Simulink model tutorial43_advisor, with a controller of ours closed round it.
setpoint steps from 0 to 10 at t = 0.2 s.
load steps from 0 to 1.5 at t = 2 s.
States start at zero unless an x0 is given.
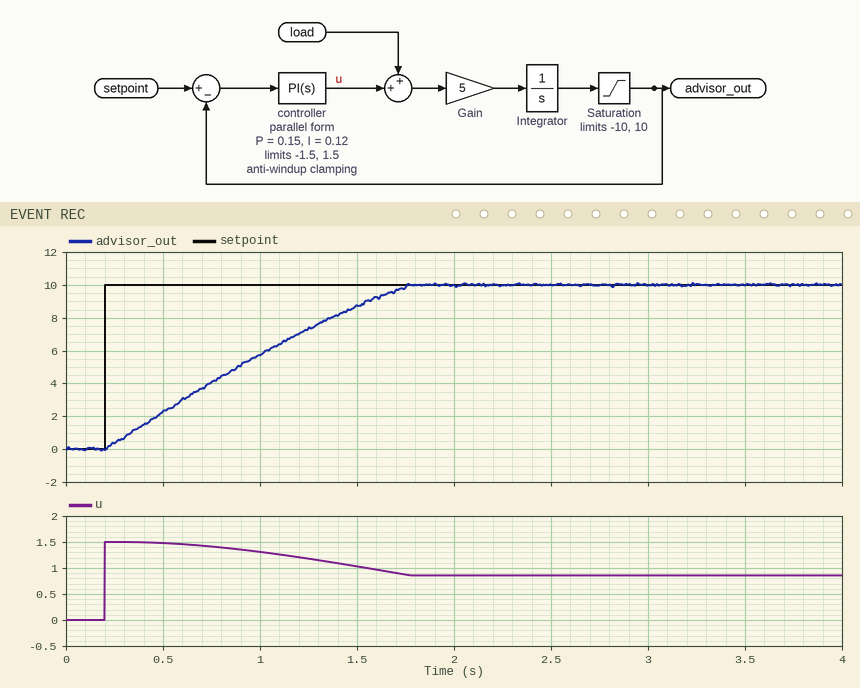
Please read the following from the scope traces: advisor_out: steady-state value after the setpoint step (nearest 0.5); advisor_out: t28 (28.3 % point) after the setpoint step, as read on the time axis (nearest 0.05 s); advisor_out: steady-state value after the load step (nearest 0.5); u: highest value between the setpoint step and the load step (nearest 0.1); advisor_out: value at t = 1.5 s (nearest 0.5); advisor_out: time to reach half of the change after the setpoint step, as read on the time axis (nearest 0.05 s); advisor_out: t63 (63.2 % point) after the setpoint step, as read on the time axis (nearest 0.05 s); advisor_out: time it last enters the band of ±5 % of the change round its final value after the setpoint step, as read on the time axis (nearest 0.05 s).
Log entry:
10.0
0.60 s
10.0
1.5
8.5
0.90 s
1.10 s
1.65 s
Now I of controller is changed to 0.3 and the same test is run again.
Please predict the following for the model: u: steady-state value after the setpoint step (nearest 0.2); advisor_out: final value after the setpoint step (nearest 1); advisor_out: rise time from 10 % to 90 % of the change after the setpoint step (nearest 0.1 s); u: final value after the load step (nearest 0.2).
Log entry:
1.2
10
1.1 s
1.2
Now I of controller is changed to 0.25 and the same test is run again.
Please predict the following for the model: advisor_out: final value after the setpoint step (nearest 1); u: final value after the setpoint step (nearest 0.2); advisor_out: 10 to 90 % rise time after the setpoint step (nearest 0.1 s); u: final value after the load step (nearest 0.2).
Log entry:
10
1.2
1.1 s
1.2
